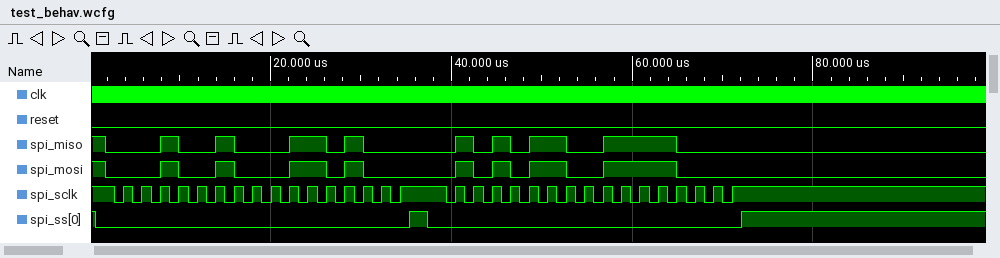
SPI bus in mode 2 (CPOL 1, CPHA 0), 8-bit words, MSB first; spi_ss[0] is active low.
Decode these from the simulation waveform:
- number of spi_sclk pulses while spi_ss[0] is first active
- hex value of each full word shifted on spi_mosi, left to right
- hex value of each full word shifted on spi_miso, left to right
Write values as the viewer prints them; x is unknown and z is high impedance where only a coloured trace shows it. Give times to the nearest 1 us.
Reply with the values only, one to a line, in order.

16
12, 34, 56, 78
12, 34, 56, 78
